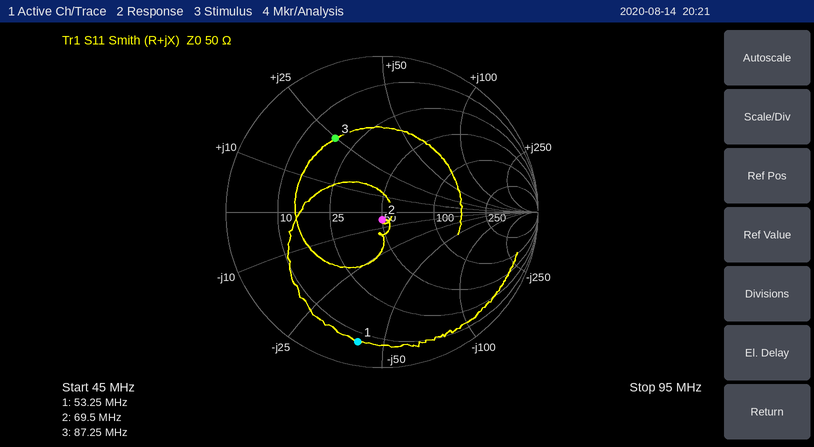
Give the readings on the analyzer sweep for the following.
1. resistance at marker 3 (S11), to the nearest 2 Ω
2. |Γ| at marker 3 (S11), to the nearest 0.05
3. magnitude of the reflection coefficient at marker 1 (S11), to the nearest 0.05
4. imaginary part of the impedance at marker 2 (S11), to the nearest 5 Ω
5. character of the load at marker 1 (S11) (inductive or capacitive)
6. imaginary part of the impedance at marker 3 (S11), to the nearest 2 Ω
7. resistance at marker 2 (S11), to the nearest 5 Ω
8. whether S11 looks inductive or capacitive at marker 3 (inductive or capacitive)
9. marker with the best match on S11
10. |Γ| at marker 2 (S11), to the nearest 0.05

18 Ω
0.55
0.85
-5 Ω
capacitive
+24 Ω
50 Ω
inductive
marker 2
0.05
